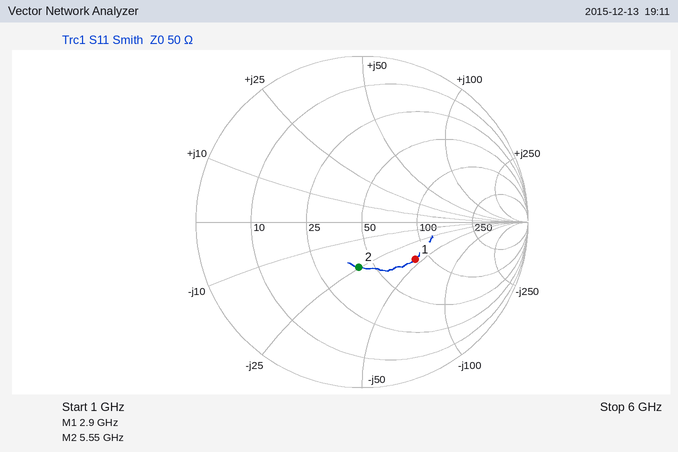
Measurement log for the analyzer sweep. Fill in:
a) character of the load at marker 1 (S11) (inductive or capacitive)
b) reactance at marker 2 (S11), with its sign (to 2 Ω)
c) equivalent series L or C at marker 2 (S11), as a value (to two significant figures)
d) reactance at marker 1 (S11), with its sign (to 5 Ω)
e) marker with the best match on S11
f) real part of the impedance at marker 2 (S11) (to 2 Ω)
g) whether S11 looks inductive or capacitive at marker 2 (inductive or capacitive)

capacitive
-24 Ω
1.2 pF
-45 Ω
marker 2
42 Ω
capacitive
